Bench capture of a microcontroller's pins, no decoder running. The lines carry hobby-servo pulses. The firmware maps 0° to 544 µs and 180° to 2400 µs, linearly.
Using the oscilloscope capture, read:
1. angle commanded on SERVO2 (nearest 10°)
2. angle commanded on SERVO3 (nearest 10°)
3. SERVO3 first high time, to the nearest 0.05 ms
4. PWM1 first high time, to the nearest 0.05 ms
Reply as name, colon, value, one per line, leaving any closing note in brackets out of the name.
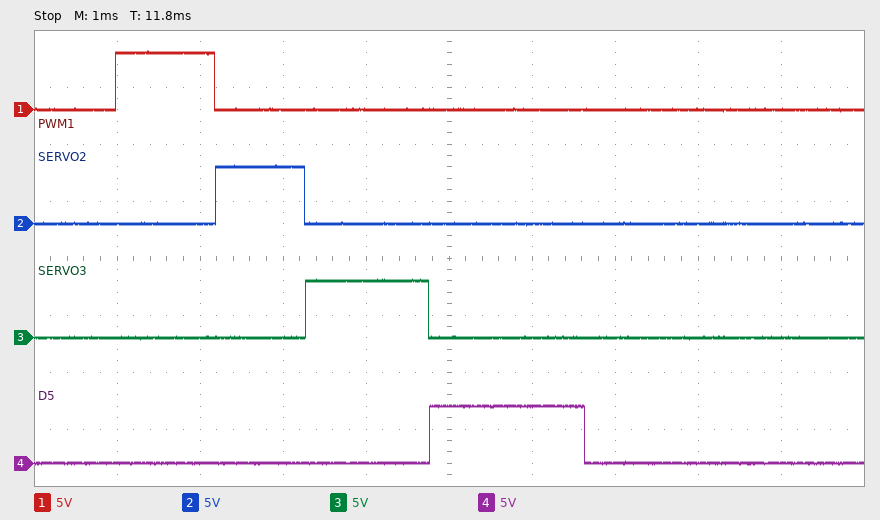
angle commanded on SERVO2: 50°
angle commanded on SERVO3: 90°
SERVO3 first high time, to the nearest 0.05 ms: 1.50 ms
PWM1 first high time, to the nearest 0.05 ms: 1.20 ms
